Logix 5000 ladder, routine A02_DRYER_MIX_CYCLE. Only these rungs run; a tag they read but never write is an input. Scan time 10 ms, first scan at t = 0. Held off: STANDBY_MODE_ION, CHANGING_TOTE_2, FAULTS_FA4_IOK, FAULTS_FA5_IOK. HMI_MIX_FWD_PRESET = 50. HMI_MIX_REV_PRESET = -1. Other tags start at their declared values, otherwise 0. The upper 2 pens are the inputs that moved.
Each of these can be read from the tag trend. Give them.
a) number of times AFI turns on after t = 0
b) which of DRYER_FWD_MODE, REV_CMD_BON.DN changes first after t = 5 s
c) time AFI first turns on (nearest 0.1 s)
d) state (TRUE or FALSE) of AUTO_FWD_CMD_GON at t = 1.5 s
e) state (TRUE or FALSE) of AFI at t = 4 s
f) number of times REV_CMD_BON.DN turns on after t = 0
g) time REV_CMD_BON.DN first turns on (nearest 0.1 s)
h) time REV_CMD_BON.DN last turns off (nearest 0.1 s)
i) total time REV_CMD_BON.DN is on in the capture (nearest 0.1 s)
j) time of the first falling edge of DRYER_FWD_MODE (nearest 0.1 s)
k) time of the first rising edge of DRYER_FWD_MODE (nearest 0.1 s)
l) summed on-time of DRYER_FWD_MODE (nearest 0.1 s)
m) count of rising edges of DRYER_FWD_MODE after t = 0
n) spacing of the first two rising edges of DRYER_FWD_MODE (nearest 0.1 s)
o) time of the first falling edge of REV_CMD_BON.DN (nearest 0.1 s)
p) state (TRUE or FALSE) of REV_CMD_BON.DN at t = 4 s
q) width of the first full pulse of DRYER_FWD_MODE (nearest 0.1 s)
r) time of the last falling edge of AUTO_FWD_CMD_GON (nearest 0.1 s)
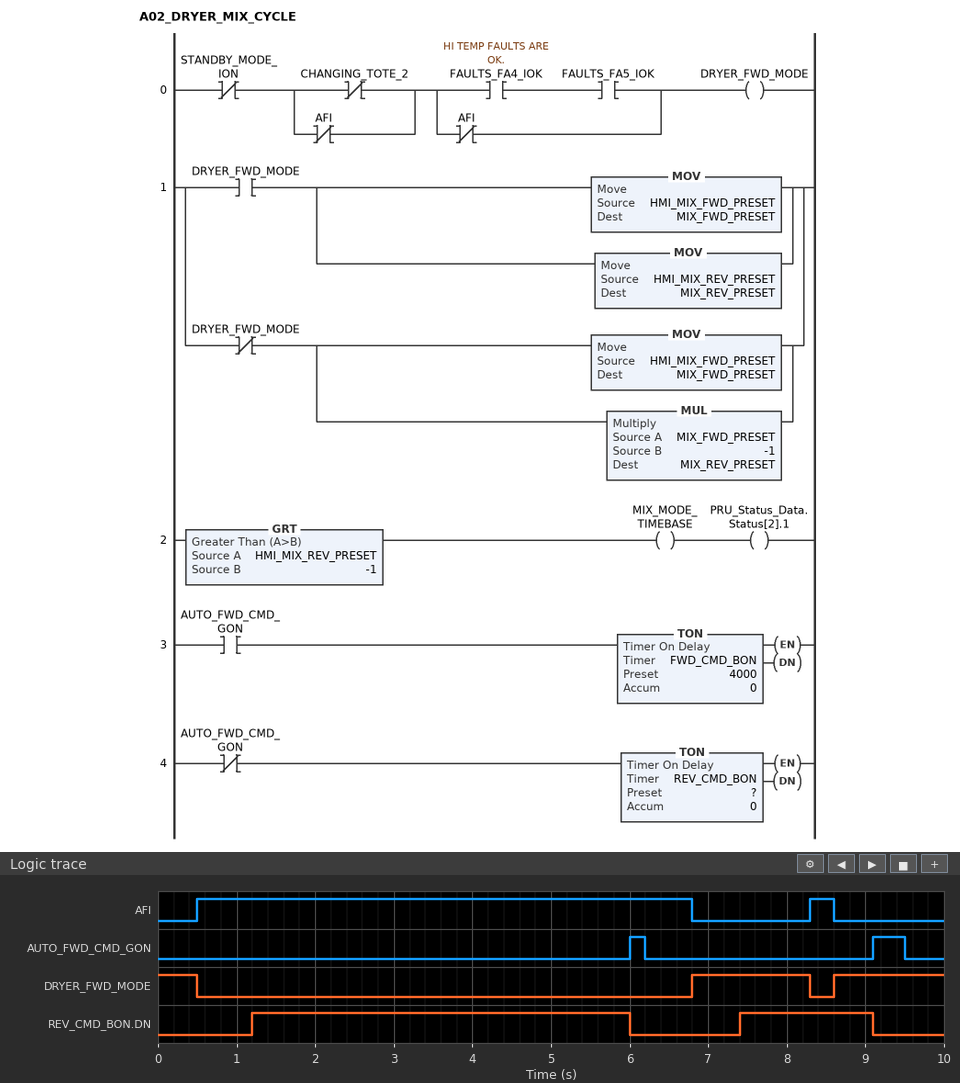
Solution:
2
REV_CMD_BON.DN
0.5 s
FALSE
TRUE
2
1.2 s
9.1 s
6.5 s
0.5 s
6.8 s
3.4 s
2
1.8 s
6.0 s
TRUE
1.5 s
9.5 s
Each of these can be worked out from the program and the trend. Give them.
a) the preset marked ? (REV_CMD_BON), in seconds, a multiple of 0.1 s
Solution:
1.2 s
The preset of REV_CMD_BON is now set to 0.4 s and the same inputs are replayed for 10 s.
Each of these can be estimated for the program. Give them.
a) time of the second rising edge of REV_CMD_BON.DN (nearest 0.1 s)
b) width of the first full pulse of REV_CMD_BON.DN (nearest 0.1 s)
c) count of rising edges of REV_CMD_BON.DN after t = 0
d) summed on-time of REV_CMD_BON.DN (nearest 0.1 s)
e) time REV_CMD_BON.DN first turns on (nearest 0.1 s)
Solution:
6.6 s
5.6 s
3
8.2 s
0.4 s
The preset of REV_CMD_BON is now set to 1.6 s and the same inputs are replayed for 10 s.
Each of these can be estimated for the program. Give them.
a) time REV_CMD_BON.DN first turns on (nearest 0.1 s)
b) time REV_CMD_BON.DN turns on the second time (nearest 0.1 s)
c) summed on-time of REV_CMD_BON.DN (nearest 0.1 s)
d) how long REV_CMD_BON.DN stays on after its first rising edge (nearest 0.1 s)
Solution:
1.6 s
7.8 s
5.7 s
4.4 s
